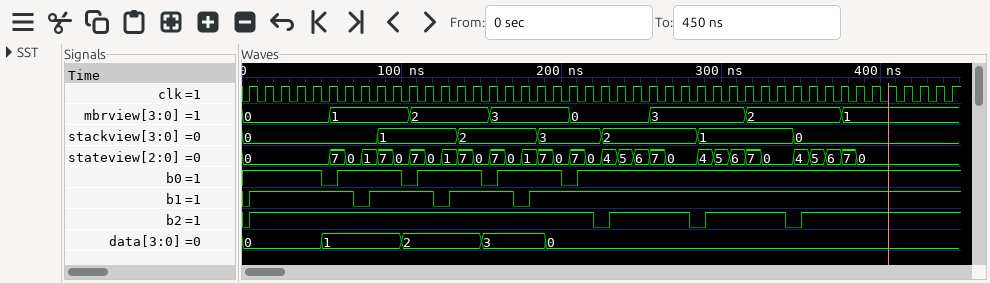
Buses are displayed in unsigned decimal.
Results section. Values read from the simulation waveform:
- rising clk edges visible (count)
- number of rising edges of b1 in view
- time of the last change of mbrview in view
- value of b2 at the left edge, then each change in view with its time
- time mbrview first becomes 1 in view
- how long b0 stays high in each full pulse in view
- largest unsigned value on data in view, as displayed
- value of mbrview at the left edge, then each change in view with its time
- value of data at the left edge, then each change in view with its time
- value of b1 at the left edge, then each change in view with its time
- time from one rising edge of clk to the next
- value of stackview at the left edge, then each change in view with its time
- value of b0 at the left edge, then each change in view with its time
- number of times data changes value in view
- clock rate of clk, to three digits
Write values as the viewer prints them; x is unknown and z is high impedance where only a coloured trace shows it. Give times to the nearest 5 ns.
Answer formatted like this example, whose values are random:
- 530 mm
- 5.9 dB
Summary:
- 45
- 4
- 375 ns
- 0, 1 at 5 ns, 0 at 220 ns, 1 at 230 ns, 0 at 280 ns, 1 at 290 ns, 0 at 340 ns, 1 at 350 ns
- 55 ns
- 40 ns, 40 ns, 40 ns
- 3
- 0, 1 at 55 ns, 2 at 105 ns, 3 at 155 ns, 0 at 205 ns, 3 at 255 ns, 2 at 315 ns, 1 at 375 ns
- 0, 1 at 50 ns, 2 at 100 ns, 3 at 150 ns, 0 at 190 ns
- 0, 1 at 5 ns, 0 at 70 ns, 1 at 80 ns, 0 at 120 ns, 1 at 130 ns, 0 at 170 ns, 1 at 180 ns
- 10 ns
- 0, 1 at 85 ns, 2 at 135 ns, 3 at 185 ns, 2 at 225 ns, 1 at 285 ns, 0 at 345 ns
- 1, 0 at 50 ns, 1 at 60 ns, 0 at 100 ns, 1 at 110 ns, 0 at 150 ns, 1 at 160 ns, 0 at 200 ns, 1 at 210 ns
- 4
- 100 MHz
